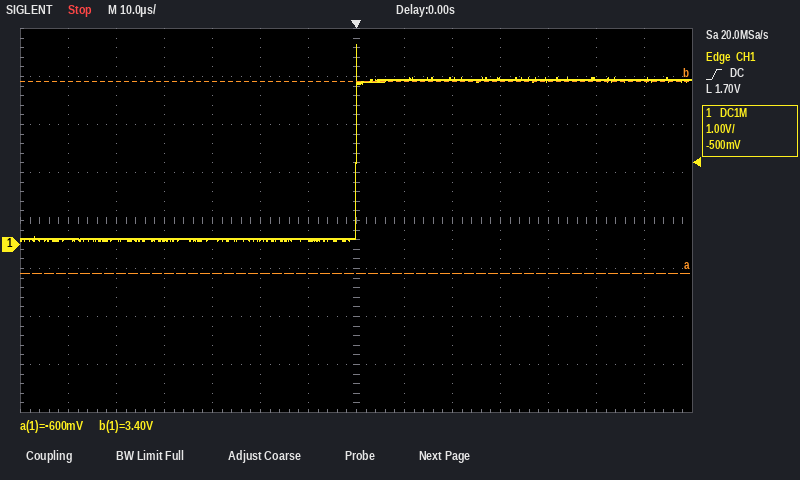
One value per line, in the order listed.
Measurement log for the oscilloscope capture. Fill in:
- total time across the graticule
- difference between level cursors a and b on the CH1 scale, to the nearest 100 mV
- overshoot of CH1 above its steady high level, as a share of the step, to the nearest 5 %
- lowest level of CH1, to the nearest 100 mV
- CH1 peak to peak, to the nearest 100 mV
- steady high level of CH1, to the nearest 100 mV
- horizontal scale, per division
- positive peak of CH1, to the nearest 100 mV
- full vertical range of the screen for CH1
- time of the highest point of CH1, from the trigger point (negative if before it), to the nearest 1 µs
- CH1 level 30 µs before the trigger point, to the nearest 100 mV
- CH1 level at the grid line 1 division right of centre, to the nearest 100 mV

140 µs
4.0 V
20 %
100 mV
4.1 V
3.4 V
10 µs
4.2 V
8 V
0 µs
100 mV
3.4 V
